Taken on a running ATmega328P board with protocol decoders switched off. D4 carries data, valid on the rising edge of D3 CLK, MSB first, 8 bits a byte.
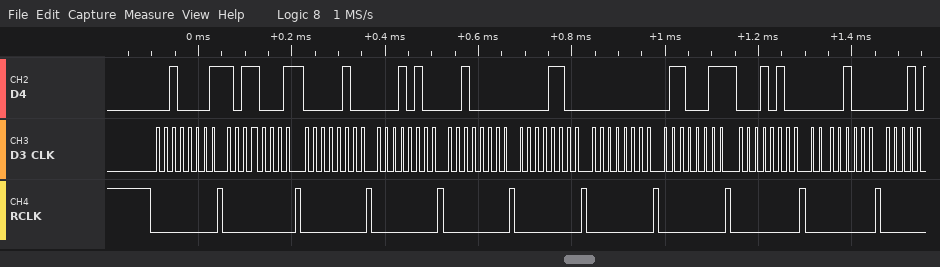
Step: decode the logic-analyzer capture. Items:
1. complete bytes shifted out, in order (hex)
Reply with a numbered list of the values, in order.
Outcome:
1. 0x21 0xB1 0x04 0x14 0x20 0x0C 0x00 0x63 0x14 0x08
